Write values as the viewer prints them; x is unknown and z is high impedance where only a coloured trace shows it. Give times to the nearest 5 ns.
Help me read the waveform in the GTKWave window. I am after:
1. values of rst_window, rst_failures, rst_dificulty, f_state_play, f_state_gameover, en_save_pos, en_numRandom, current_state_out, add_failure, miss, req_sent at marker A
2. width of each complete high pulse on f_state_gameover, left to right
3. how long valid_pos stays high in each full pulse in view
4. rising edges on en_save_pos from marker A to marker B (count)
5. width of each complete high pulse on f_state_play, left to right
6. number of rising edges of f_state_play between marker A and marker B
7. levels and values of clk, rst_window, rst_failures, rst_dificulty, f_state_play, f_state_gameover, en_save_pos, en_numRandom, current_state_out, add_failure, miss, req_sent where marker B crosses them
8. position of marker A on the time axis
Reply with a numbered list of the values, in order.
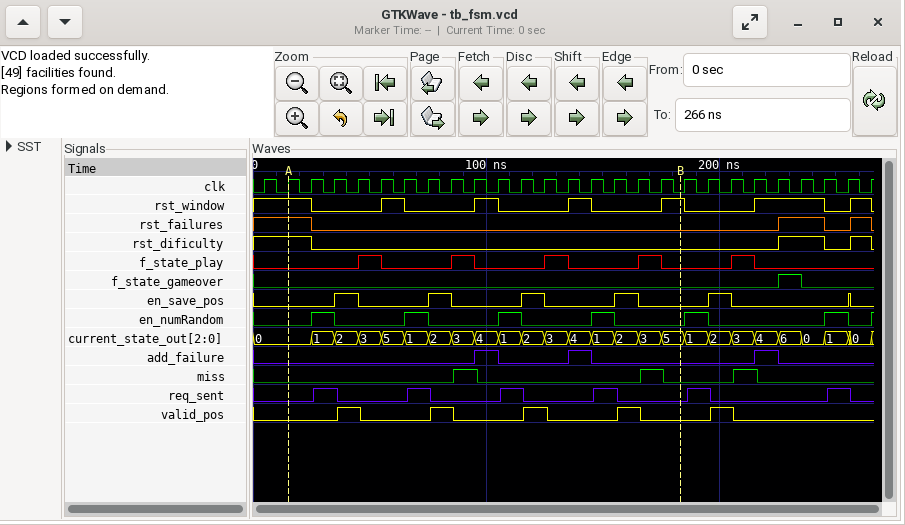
1. rst_window=1, rst_failures=1, rst_dificulty=1, f_state_play=0, f_state_gameover=0, en_save_pos=0, en_numRandom=0, current_state_out=0, add_failure=0, miss=0, req_sent=0
2. 10 ns
3. 10 ns, 10 ns, 10 ns, 10 ns, 10 ns
4. 4
5. 10 ns, 10 ns, 10 ns, 10 ns, 10 ns
6. 4
7. clk=0, rst_window=1, rst_failures=0, rst_dificulty=0, f_state_play=0, f_state_gameover=0, en_save_pos=0, en_numRandom=0, current_state_out=5, add_failure=0, miss=0, req_sent=0
8. 15 ns
